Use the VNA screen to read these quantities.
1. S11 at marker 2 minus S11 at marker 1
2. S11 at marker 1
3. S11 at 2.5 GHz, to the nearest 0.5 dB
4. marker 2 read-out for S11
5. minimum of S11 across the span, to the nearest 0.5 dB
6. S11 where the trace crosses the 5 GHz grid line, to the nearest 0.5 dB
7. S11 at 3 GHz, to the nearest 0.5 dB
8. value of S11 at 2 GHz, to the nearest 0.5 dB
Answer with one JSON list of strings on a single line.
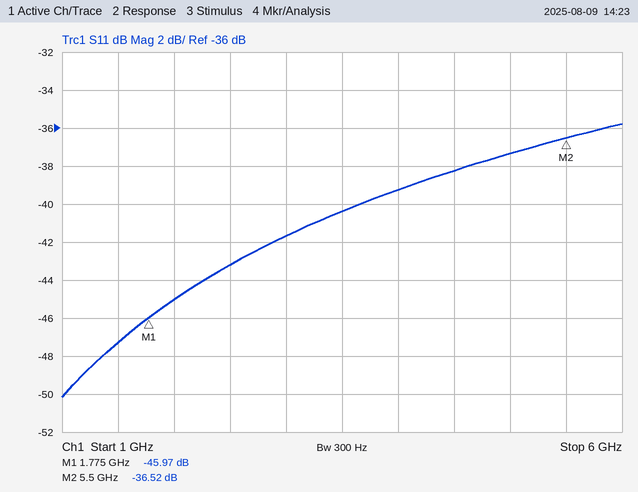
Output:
["9.45 dB", "-45.97 dB", "-43.0 dB", "-36.52 dB", "-50.0 dB", "-37.5 dB", "-41.5 dB", "-45.0 dB"]
